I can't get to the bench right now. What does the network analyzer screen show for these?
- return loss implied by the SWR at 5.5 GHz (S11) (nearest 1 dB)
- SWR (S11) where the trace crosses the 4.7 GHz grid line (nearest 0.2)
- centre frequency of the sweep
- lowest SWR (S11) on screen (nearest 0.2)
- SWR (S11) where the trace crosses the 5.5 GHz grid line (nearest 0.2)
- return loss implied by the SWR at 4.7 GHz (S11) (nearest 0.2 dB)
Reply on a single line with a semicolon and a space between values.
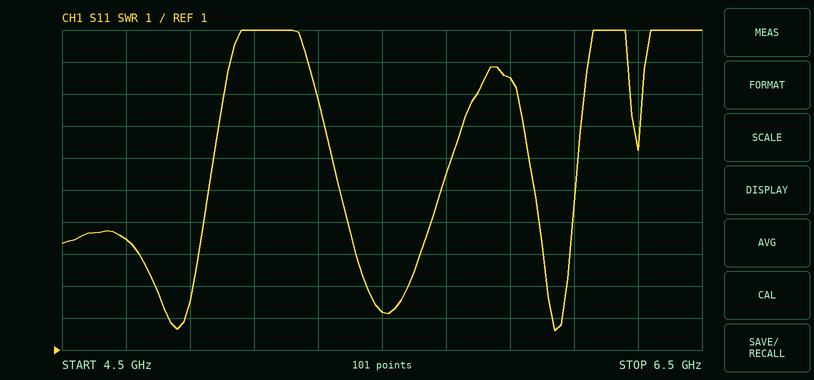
9 dB; 4.4; 5.5 GHz; 1.6; 2.2; 4.0 dB
